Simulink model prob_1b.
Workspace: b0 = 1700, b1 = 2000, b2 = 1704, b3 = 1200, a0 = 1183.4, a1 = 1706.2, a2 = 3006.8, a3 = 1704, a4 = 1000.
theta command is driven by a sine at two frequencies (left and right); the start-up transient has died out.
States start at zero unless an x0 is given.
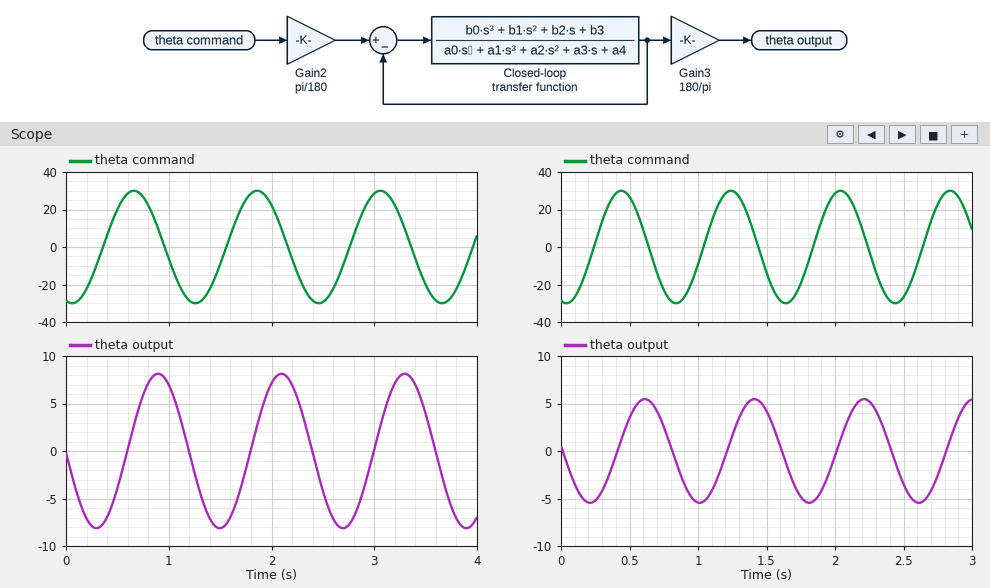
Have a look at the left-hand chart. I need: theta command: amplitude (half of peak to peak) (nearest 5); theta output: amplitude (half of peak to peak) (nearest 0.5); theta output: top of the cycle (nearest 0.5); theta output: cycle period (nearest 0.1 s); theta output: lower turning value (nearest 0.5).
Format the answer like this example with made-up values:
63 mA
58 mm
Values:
30
8.0
8.0
1.2 s
-8.0
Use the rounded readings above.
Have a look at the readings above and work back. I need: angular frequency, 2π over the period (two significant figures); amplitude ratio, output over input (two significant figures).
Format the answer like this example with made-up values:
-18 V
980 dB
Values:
5.2 rad/s
0.27
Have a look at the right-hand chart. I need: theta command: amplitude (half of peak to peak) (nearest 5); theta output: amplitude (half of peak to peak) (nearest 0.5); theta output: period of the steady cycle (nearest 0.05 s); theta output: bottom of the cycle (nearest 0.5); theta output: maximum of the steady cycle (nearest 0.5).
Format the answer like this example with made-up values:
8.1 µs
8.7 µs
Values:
30
5.5
0.80 s
-5.5
5.5
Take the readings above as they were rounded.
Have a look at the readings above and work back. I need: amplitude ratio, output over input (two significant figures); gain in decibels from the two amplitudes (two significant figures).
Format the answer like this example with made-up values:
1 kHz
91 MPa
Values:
0.18
-15 dB
